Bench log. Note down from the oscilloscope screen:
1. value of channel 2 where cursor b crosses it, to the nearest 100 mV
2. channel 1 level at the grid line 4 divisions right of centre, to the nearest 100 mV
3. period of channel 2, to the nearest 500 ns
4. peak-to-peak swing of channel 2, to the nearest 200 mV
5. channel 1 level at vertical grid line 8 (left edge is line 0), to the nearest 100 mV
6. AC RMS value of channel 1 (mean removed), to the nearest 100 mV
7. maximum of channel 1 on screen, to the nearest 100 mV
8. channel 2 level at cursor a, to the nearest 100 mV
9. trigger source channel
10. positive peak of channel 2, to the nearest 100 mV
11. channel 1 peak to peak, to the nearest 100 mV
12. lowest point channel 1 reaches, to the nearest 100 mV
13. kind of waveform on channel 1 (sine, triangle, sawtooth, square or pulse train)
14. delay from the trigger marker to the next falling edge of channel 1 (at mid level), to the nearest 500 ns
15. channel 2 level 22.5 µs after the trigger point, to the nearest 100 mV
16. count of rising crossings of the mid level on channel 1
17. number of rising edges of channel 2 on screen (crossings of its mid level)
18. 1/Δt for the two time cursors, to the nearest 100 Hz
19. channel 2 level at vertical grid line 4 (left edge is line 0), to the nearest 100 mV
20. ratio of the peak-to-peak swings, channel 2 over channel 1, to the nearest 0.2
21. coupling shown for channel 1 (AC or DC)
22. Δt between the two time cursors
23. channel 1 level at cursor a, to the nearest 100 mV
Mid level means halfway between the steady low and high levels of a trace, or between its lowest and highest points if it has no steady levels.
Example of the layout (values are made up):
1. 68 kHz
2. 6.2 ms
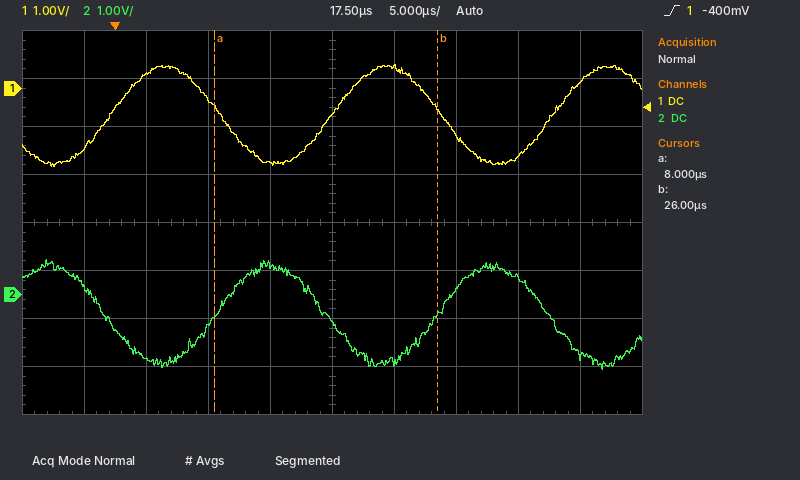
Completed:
1. -400 mV
2. 100 mV
3. 18.0 µs
4. 2.2 V
5. -1.4 V
6. 700 mV
7. 500 mV
8. -500 mV
9. channel 1
10. 700 mV
11. 2.1 V
12. -1.6 V
13. sine
14. 8.5 µs
15. -1.4 V
16. 3
17. 2
18. 55.6 kHz
19. 600 mV
20. 1.0
21. DC
22. 18.0 µs
23. -400 mV
